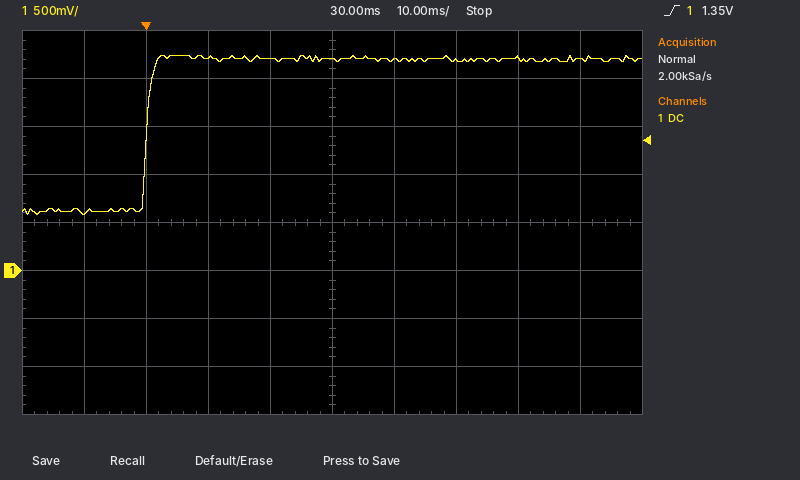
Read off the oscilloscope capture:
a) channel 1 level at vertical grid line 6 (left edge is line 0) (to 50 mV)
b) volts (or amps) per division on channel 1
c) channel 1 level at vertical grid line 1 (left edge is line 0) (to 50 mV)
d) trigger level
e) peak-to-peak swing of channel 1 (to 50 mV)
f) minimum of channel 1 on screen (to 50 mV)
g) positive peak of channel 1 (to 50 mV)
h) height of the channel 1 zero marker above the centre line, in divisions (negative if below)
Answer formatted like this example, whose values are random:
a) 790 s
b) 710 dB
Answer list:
a) 2.20 V
b) 500 mV
c) 600 mV
d) 1.35 V
e) 1.65 V
f) 600 mV
g) 2.25 V
h) -1.0 div
